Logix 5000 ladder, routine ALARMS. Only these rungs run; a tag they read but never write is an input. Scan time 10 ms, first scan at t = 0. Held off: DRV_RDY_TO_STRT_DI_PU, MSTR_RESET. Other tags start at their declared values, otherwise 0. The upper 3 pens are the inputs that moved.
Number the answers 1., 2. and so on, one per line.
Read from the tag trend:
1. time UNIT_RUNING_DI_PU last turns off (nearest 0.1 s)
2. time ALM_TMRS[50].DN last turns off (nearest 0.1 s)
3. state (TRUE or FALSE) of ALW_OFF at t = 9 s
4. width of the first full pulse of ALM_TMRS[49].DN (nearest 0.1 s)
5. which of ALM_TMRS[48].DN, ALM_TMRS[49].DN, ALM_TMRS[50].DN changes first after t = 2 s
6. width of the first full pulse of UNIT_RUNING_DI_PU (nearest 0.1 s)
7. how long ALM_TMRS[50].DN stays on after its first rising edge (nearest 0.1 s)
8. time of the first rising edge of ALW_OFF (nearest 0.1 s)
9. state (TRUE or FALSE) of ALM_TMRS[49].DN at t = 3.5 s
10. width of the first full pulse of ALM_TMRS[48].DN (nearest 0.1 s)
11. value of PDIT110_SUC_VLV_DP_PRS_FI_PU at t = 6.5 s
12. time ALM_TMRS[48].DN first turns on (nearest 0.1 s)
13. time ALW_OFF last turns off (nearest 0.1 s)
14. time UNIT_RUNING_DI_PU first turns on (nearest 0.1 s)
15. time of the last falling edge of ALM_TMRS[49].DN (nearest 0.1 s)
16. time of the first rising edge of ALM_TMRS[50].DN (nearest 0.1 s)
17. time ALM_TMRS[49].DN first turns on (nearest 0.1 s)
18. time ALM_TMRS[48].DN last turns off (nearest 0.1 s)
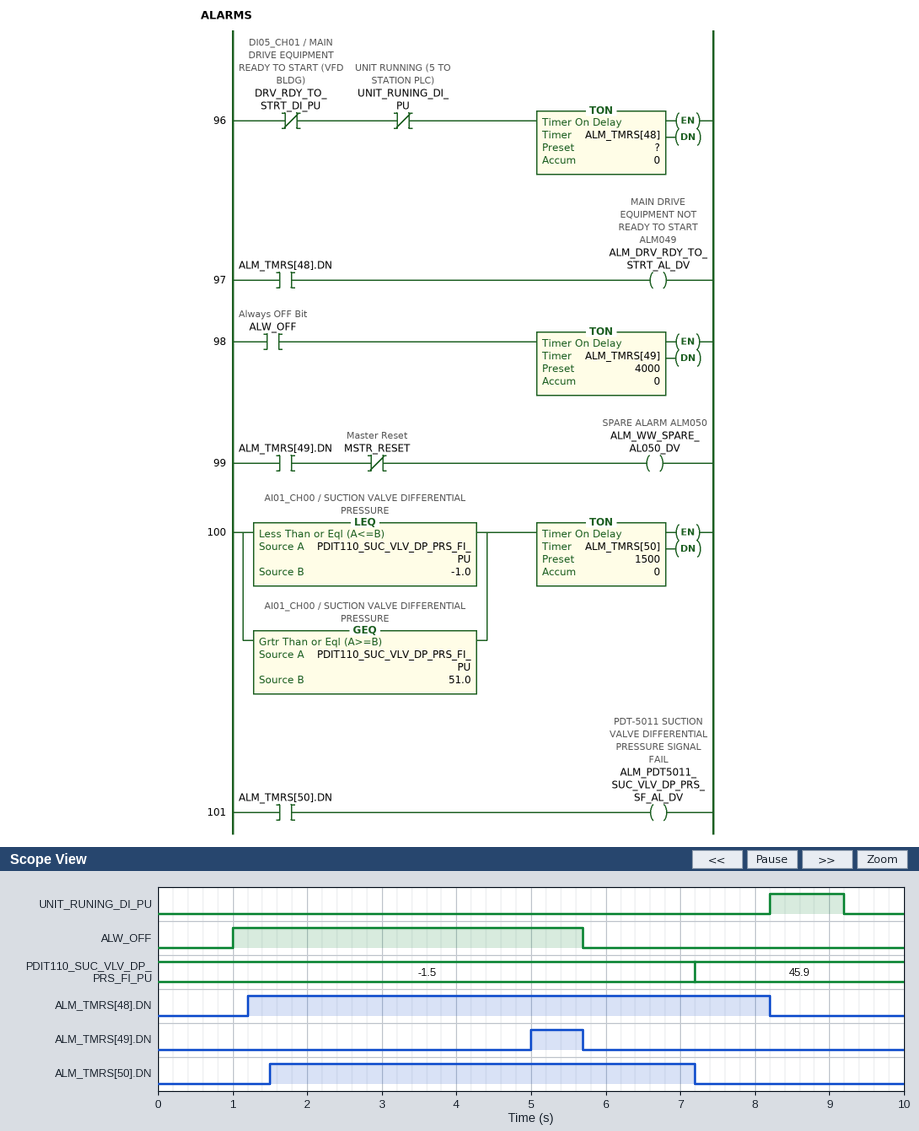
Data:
1. 9.2 s
2. 7.2 s
3. FALSE
4. 0.7 s
5. ALM_TMRS[49].DN
6. 1.0 s
7. 5.7 s
8. 1.0 s
9. FALSE
10. 7.0 s
11. -1.5
12. 1.2 s
13. 5.7 s
14. 8.2 s
15. 5.7 s
16. 1.5 s
17. 5.0 s
18. 8.2 s
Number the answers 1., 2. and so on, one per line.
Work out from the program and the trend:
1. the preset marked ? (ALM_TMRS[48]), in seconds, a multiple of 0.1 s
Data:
1. 1.2 s
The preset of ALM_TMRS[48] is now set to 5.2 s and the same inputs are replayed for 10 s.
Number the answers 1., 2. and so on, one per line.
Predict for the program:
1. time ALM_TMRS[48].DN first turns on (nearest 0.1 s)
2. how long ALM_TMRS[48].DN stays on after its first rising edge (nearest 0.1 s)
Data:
1. 5.2 s
2. 3.0 s
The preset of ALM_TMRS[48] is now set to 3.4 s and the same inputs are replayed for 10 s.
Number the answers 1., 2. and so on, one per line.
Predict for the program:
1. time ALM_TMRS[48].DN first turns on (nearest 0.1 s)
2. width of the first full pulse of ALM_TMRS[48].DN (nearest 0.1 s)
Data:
1. 3.4 s
2. 4.8 s
